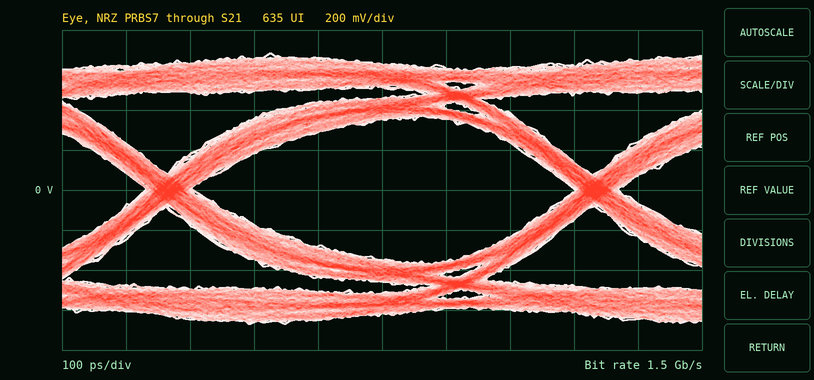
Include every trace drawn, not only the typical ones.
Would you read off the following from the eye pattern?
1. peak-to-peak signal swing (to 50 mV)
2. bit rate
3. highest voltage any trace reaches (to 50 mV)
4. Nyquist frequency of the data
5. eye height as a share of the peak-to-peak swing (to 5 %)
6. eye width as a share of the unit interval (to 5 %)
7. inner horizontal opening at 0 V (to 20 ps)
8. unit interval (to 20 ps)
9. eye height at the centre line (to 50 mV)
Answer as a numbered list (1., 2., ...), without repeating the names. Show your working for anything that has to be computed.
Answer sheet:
1. 1.35 V
2. 1.5 Gb/s
3. 700 mV
4. 750 MHz
5. 700 mV / 1.35 V ≈ 51.9 %, so 50 % to the nearest 5 %
6. 600 ps / 660 ps ≈ 90.9 %, so 90 % to the nearest 5 %
7. 600 ps
8. 660 ps
9. 700 mV
